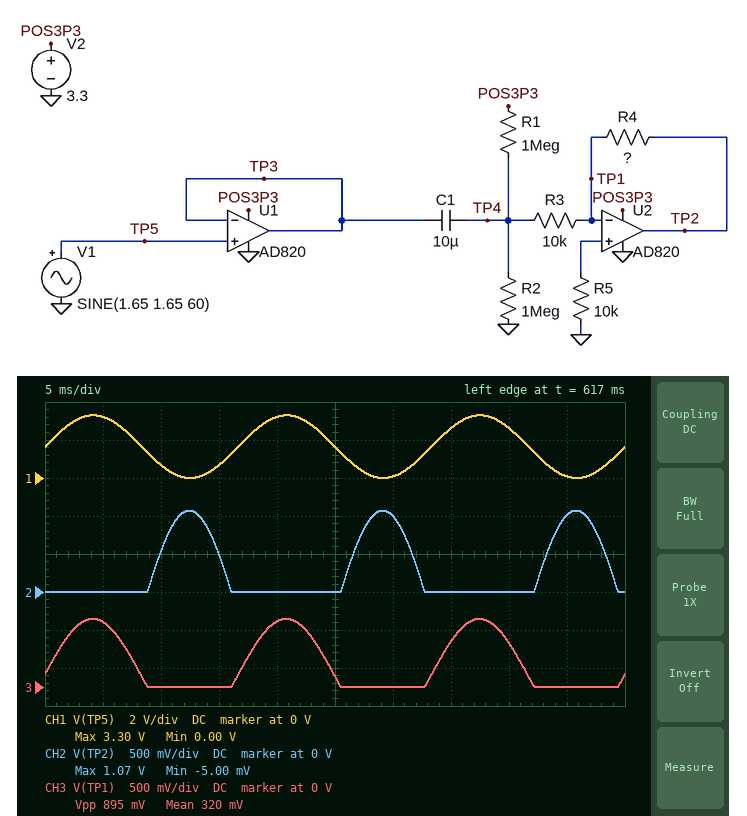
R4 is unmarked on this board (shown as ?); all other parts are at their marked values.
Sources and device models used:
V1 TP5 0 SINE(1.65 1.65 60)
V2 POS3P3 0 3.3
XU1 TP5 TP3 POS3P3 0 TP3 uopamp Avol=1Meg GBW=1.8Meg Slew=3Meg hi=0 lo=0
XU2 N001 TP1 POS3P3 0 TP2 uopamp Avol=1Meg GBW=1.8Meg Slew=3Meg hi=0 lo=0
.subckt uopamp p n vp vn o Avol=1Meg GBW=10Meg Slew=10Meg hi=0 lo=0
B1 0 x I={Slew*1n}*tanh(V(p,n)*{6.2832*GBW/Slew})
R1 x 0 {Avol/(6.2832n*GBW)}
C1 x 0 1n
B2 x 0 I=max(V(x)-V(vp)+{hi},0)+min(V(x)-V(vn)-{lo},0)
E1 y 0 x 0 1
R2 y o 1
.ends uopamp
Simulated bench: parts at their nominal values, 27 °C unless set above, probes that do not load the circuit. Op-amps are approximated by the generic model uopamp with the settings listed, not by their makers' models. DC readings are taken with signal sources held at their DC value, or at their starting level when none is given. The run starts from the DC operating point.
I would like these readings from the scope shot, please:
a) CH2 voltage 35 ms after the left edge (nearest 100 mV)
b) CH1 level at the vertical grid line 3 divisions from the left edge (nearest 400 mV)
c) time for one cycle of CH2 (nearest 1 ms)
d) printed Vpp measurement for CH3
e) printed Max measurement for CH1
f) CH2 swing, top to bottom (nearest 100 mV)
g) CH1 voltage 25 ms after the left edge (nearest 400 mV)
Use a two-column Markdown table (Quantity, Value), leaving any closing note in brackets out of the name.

| Quantity | Value |
|---|---|
| CH2 voltage 35 ms after the left edge | 0 V |
| CH1 level at the vertical grid line 3 divisions from the left edge | 800 mV |
| time for one cycle of CH2 | 17 ms |
| printed Vpp measurement for CH3 | 895 mV |
| printed Max measurement for CH1 | 3.30 V |
| CH2 swing, top to bottom | 1.1 V |
| CH1 voltage 25 ms after the left edge | 1.6 V |
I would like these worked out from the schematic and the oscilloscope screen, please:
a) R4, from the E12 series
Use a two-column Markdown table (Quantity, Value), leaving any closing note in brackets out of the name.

| Quantity | Value |
|---|---|
| R4, from the E12 series | 8.2 kΩ |
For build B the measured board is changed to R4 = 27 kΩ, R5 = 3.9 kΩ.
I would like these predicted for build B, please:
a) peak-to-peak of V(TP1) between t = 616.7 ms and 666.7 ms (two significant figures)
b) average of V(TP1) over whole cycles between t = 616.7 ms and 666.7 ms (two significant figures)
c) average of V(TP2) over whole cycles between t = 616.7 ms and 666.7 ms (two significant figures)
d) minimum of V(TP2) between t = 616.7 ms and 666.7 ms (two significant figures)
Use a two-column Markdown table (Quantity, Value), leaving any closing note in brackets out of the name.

| Quantity | Value |
|---|---|
| peak-to-peak of V(TP1) between t = 616.7 ms and 666.7 ms | 1.7 V |
| average of V(TP1) over whole cycles between t = 616.7 ms and 666.7 ms | 660 mV |
| average of V(TP2) over whole cycles between t = 616.7 ms and 666.7 ms | 630 mV |
| minimum of V(TP2) between t = 616.7 ms and 666.7 ms | -3.0 mV |
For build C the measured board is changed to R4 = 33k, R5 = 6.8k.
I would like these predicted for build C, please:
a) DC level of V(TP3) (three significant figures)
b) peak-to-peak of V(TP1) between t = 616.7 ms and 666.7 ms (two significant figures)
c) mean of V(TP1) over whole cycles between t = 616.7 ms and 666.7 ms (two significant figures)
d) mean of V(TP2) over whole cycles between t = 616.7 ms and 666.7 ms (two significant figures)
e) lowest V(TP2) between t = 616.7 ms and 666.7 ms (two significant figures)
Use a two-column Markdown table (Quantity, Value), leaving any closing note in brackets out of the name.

| Quantity | Value |
|---|---|
| DC level of V(TP3) | 1.65 V |
| peak-to-peak of V(TP1) between t = 616.7 ms and 666.7 ms | 1.8 V |
| mean of V(TP1) over whole cycles between t = 616.7 ms and 666.7 ms | 720 mV |
| mean of V(TP2) over whole cycles between t = 616.7 ms and 666.7 ms | 700 mV |
| lowest V(TP2) between t = 616.7 ms and 666.7 ms | -3.0 mV |
